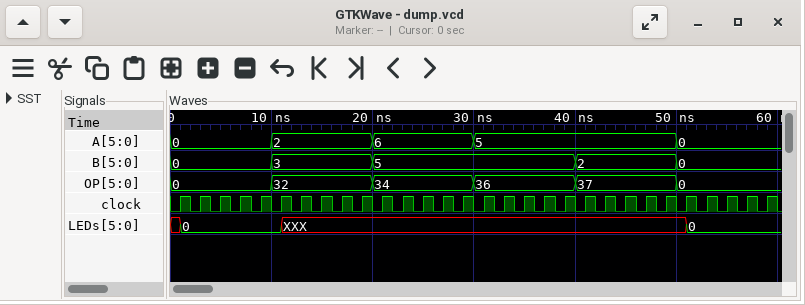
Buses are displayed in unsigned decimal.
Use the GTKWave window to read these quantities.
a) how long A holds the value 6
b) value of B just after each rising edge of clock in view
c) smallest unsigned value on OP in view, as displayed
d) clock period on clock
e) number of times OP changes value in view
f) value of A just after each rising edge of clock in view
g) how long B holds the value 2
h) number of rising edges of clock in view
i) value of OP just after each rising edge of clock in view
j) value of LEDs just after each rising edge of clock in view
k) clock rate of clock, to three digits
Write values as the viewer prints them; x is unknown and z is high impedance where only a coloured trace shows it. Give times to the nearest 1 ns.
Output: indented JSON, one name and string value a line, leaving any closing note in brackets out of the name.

{
  "how long A holds the value 6": "10 ns",
  "value of B just after each rising edge of clock in view": "0, 0, 0, 0, 0, 3, 3, 3, 3, 3, 5, 5, 5, 5, 5, 5, 5, 5, 5, 5, 2, 2, 2, 2, 2, 0, 0, 0, 0, 0",
  "smallest unsigned value on OP in view, as displayed": "0",
  "clock period on clock": "2 ns",
  "number of times OP changes value in view": "5",
  "value of A just after each rising edge of clock in view": "0, 0, 0, 0, 0, 2, 2, 2, 2, 2, 6, 6, 6, 6, 6, 5, 5, 5, 5, 5, 5, 5, 5, 5, 5, 0, 0, 0, 0, 0",
  "how long B holds the value 2": "10 ns",
  "number of rising edges of clock in view": "30",
  "value of OP just after each rising edge of clock in view": "0, 0, 0, 0, 0, 32, 32, 32, 32, 32, 34, 34, 34, 34, 34, 36, 36, 36, 36, 36, 37, 37, 37, 37, 37, 0, 0, 0, 0, 0",
  "value of LEDs just after each rising edge of clock in view": "0, 0, 0, 0, 0, XXX, XXX, XXX, XXX, XXX, XXX, XXX, XXX, XXX, XXX, XXX, XXX, XXX, XXX, XXX, XXX, XXX, XXX, XXX, XXX, 0, 0, 0, 0, 0",
  "clock rate of clock, to three digits": "500 MHz"
}
